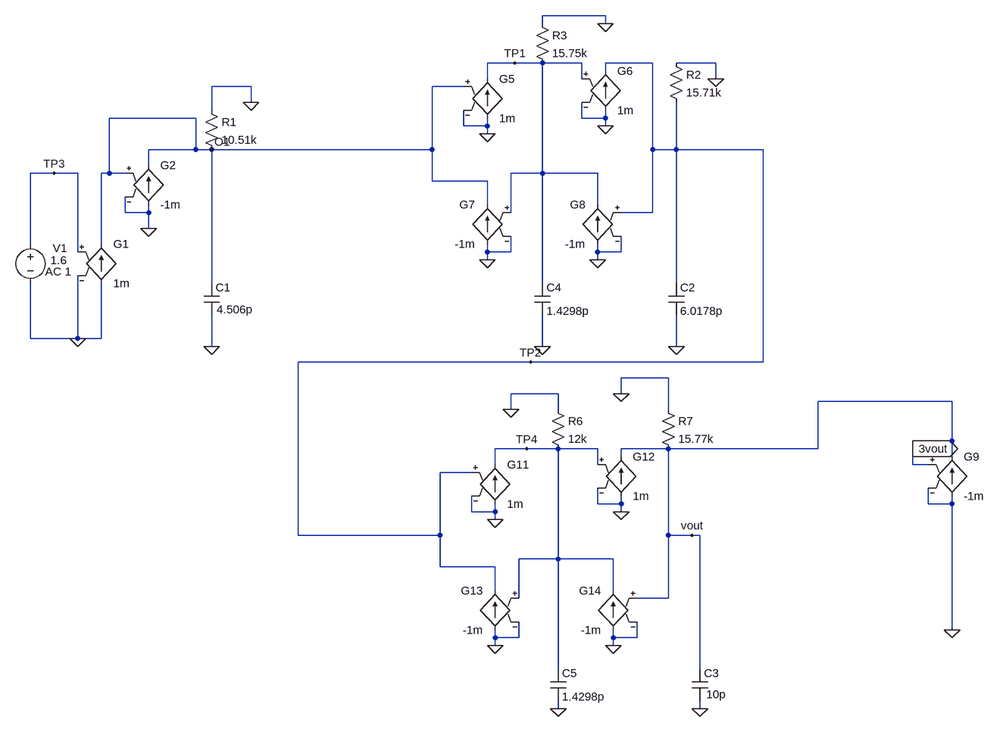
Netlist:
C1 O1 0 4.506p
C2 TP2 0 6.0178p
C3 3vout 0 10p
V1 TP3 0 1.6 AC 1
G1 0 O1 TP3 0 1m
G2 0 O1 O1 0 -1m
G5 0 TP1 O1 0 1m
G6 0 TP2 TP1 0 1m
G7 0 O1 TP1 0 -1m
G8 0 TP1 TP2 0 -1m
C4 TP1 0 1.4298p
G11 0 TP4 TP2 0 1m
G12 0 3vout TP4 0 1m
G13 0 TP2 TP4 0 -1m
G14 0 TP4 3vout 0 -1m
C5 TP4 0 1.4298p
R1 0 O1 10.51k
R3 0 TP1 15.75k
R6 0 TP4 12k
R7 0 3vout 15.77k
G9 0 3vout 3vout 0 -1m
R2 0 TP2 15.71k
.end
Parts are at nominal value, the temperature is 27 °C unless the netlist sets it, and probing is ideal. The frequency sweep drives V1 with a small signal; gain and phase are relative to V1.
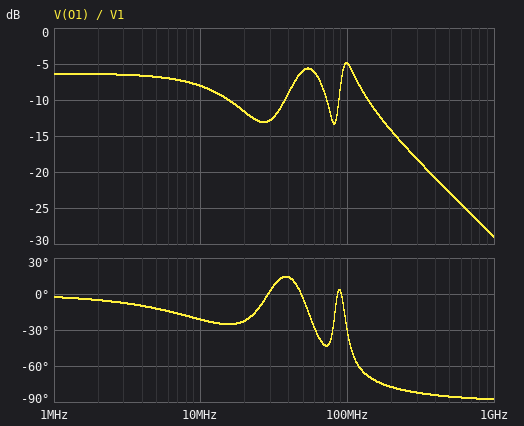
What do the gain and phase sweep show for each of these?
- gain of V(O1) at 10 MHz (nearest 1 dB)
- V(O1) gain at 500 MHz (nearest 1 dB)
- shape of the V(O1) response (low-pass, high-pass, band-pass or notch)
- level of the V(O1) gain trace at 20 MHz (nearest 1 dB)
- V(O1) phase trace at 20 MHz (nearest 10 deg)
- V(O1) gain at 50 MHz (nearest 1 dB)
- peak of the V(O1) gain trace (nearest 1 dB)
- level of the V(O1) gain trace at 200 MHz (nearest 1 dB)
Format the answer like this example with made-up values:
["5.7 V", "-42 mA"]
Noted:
["-8 dB", "-23 dB", "low-pass", "-12 dB", "-20 deg", "-6 dB", "-5 dB", "-14 dB"]
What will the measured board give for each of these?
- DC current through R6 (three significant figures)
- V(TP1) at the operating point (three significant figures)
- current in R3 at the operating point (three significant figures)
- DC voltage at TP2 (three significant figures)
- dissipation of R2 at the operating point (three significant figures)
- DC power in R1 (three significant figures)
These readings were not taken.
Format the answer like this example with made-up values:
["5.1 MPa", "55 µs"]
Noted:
["59.0 µA", "754 mV", "47.9 µA", "725 mV", "33.4 µW", "56.8 µW"]
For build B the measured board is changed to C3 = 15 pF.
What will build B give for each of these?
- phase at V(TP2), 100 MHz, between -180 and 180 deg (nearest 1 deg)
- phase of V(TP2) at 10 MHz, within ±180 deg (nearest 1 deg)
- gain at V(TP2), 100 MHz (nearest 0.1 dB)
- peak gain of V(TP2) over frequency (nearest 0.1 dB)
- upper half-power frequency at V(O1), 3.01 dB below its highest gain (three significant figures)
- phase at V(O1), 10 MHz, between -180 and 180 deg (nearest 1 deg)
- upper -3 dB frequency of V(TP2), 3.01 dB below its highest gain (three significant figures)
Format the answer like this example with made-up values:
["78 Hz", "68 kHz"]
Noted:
["163 deg", "-35 deg", "-7.1 dB", "-3.6 dB", "118 MHz", "-24 deg", "99.0 MHz"]
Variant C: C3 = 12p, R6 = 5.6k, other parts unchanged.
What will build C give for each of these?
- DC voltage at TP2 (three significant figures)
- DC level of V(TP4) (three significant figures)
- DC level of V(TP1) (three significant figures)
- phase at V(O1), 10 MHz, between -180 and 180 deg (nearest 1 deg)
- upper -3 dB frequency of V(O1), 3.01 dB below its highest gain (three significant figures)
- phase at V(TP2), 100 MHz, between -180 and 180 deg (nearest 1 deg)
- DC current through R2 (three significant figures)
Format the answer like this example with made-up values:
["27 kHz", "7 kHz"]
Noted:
["755 mV", "675 mV", "723 mV", "-22 deg", "122 MHz", "168 deg", "48.1 µA"]
